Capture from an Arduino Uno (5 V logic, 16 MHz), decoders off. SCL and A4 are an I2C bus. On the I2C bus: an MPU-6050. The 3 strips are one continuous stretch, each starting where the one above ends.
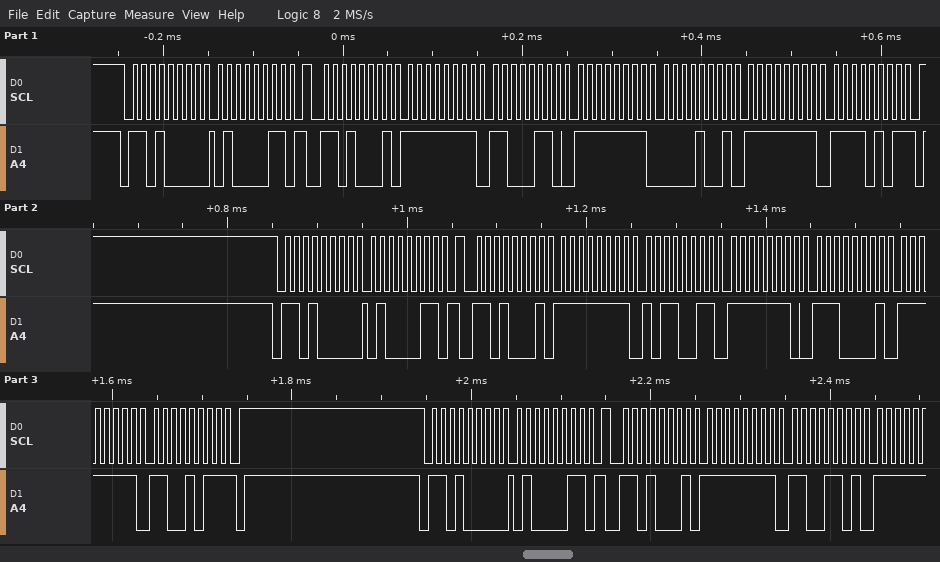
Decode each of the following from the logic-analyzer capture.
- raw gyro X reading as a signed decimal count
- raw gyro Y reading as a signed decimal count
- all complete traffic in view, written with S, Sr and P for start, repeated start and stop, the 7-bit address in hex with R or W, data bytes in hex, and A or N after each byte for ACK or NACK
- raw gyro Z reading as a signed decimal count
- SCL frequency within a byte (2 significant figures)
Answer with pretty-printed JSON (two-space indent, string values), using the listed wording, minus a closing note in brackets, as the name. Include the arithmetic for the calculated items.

{
  "raw gyro X reading as a signed decimal count": "0xFFC6 = -58",
  "raw gyro Y reading as a signed decimal count": "0xFF09 = -247",
  "all complete traffic in view, written with S, Sr and P for start, repeated start and stop, the 7-bit address in hex with R or W, data bytes in hex, and A or N after each byte for ACK or NACK": "S 68W A 43 A Sr 68R A FF A C6 A FF A 09 A FF A F5 N P S 68W A 43 A Sr 68R A FF A B3 A FE A E1 A FF A CB N P S 68W A 43 A Sr 68R A FF A CD A",
  "raw gyro Z reading as a signed decimal count": "0xFFF5 = -11",
  "SCL frequency within a byte": "100 kHz"
}
